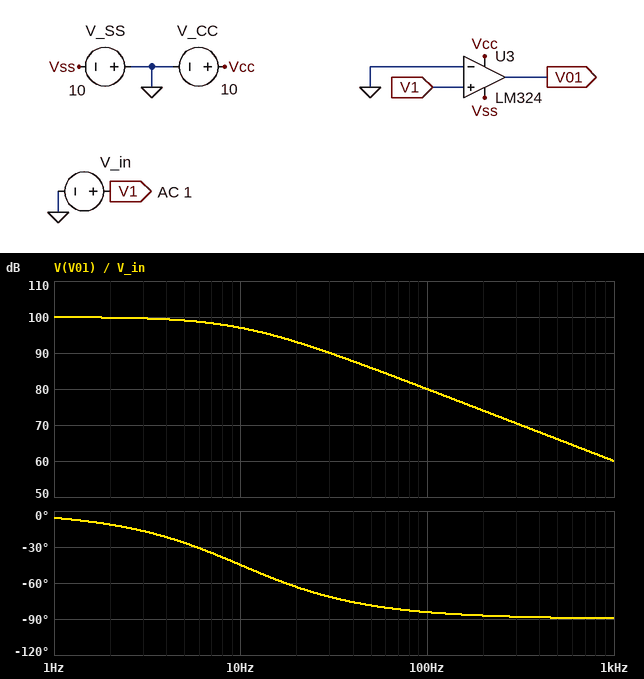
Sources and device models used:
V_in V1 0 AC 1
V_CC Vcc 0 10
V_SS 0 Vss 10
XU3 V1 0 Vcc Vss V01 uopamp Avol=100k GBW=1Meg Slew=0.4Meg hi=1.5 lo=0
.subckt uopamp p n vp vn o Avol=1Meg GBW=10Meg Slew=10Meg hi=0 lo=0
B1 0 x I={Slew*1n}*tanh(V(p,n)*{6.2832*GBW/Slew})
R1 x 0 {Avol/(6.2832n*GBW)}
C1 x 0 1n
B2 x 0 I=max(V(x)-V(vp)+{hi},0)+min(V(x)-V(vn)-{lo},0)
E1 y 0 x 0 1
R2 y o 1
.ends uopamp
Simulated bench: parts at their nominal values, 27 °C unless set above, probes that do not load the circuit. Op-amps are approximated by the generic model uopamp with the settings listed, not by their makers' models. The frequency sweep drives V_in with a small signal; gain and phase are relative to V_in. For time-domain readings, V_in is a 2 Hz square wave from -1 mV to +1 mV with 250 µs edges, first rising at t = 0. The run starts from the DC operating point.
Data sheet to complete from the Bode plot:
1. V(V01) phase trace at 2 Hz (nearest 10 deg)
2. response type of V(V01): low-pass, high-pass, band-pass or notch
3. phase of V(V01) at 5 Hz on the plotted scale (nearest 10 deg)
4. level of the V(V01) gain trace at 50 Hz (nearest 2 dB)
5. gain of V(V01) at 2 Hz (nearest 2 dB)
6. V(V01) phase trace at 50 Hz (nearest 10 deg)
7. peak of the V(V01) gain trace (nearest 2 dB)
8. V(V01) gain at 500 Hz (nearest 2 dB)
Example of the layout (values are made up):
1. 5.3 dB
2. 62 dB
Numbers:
1. -10 deg
2. low-pass
3. -30 deg
4. 86 dB
5. 100 dB
6. -80 deg
7. 100 dB
8. 66 dB
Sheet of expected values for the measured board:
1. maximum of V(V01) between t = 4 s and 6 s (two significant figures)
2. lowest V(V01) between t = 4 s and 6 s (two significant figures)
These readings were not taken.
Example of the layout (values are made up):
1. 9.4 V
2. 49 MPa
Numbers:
1. 8.5 V
2. -10 V
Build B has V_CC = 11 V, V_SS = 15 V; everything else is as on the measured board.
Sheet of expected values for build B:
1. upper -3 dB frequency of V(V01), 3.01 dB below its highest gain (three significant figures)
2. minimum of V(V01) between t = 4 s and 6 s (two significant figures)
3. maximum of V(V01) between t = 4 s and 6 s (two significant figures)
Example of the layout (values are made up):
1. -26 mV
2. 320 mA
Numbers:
1. 10.0 Hz
2. -15 V
3. 9.5 V
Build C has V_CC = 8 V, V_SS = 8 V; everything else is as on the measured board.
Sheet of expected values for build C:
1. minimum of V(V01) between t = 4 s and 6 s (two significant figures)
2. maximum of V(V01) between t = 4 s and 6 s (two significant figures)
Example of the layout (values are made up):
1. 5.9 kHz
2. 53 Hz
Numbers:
1. -8.0 V
2. 6.5 V
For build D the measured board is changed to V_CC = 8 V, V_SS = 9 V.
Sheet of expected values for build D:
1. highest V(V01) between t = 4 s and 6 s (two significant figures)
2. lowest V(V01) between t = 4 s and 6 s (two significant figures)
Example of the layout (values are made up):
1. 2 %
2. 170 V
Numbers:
1. 6.5 V
2. -9.0 V
